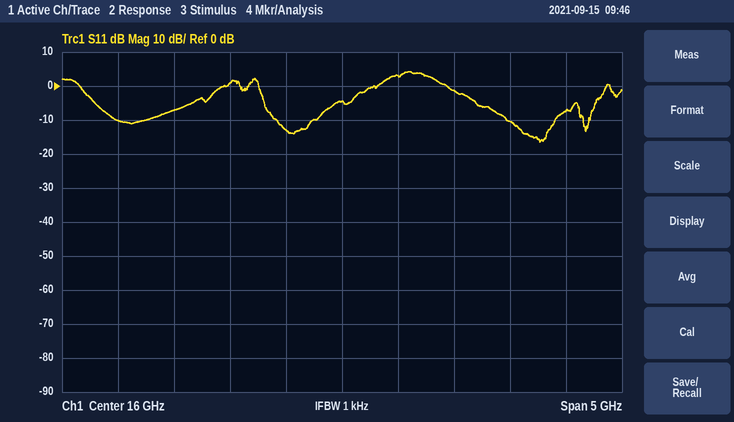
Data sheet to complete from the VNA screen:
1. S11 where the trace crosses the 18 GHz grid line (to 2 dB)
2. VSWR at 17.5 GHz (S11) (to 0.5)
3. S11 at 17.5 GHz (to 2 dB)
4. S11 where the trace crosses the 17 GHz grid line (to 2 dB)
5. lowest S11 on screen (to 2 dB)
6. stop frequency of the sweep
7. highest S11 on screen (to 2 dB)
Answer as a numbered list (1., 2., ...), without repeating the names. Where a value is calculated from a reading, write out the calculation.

1. -8 dB
2. |Γ| = 10^(-10/20) = 0.3162; VSWR = (1 + 0.3162)/(1 − 0.3162) ≈ 1.92, so 2.0 to the nearest 0.5
3. -10 dB
4. -2 dB
5. -16 dB
6. 18.5 GHz
7. 4 dB
